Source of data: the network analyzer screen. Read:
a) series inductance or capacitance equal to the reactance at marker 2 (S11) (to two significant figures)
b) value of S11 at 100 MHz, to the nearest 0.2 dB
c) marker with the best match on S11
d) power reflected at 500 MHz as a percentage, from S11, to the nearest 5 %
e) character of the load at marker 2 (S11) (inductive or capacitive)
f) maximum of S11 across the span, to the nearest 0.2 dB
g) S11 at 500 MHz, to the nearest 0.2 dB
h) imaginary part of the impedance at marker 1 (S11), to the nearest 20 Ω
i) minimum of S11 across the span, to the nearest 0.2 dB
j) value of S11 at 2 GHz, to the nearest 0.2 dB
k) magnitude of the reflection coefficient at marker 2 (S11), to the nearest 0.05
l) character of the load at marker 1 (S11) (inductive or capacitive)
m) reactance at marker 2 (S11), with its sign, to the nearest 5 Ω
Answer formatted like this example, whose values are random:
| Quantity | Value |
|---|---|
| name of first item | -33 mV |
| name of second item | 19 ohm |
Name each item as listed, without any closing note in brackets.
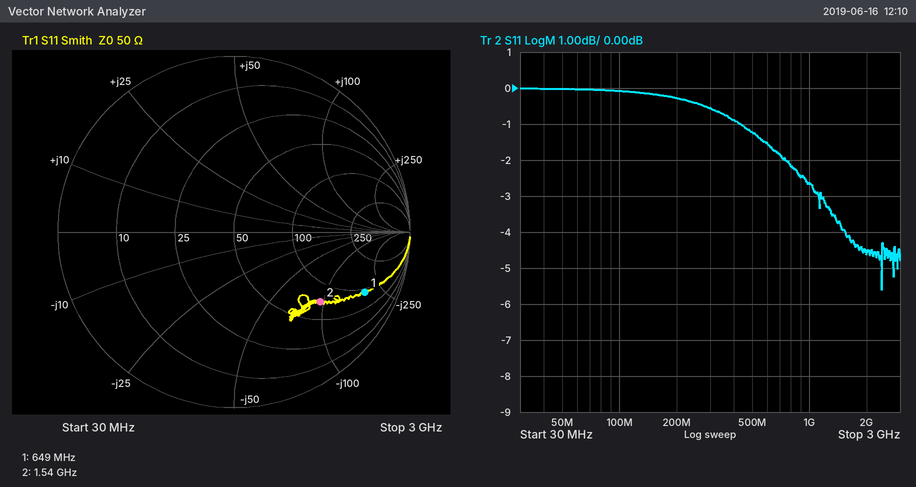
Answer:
| Quantity | Value |
|---|---|
| series inductance or capacitance equal to the reactance at marker 2 (S11) | 1.1 pF |
| value of S11 at 100 MHz, to the nearest 0.2 dB | 0.0 dB |
| marker with the best match on S11 | marker 2 |
| power reflected at 500 MHz as a percentage, from S11, to the nearest 5 % | 75 % |
| character of the load at marker 2 (S11) | capacitive |
| maximum of S11 across the span, to the nearest 0.2 dB | 0.0 dB |
| S11 at 500 MHz, to the nearest 0.2 dB | -1.2 dB |
| imaginary part of the impedance at marker 1 (S11), to the nearest 20 Ω | -180 Ω |
| minimum of S11 across the span, to the nearest 0.2 dB | -5.6 dB |
| value of S11 at 2 GHz, to the nearest 0.2 dB | -4.6 dB |
| magnitude of the reflection coefficient at marker 2 (S11), to the nearest 0.05 | 0.65 |
| character of the load at marker 1 (S11) | capacitive |
| reactance at marker 2 (S11), with its sign, to the nearest 5 Ω | -95 Ω |
